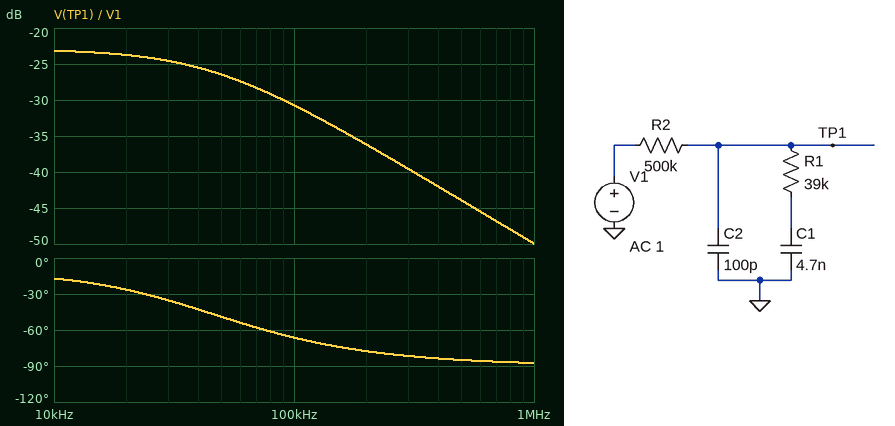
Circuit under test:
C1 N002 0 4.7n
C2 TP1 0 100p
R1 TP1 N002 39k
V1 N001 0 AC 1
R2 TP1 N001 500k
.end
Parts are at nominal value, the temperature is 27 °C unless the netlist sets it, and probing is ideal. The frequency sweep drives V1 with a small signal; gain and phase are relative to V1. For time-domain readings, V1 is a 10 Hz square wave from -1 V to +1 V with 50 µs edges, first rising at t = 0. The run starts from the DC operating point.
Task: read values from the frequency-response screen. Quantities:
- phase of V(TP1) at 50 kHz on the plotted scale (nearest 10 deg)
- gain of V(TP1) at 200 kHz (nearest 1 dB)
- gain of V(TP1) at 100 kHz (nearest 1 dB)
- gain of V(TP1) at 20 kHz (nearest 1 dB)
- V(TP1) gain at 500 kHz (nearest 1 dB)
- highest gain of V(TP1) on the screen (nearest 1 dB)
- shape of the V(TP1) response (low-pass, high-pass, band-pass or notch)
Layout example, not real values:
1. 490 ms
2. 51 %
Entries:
1. -50 deg
2. -36 dB
3. -31 dB
4. -24 dB
5. -44 dB
6. -23 dB
7. low-pass
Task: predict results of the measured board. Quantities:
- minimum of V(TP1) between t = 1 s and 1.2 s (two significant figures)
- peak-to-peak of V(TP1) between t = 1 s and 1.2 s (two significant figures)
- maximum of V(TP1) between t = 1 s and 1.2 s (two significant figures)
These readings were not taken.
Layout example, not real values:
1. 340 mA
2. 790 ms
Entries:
1. -1.0 V
2. 2.0 V
3. 1.0 V
